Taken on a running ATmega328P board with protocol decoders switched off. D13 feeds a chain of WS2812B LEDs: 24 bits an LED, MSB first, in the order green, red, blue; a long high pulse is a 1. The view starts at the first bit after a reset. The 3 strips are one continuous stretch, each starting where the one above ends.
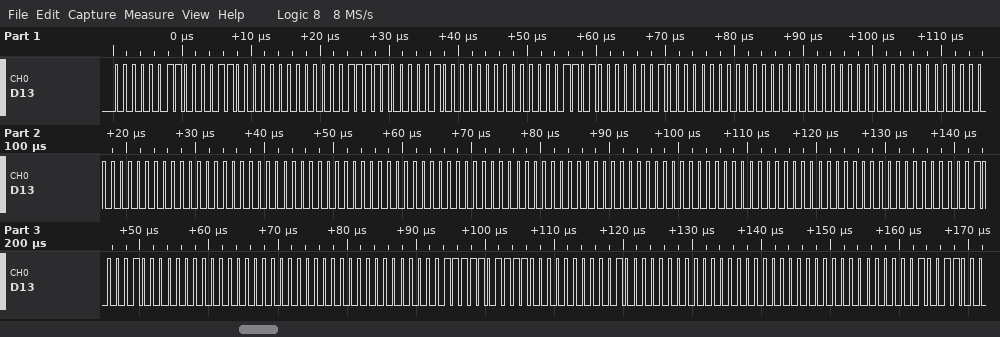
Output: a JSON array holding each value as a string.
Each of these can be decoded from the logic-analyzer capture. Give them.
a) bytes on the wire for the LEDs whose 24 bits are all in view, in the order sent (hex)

["03 0C 00 1F 04 00 0D 01 00 00 00 00 00 00 00 00 00 00 00 00 00 00 00 00 00 21 00 00 00 00 1F 78 01 00 00 00"]
